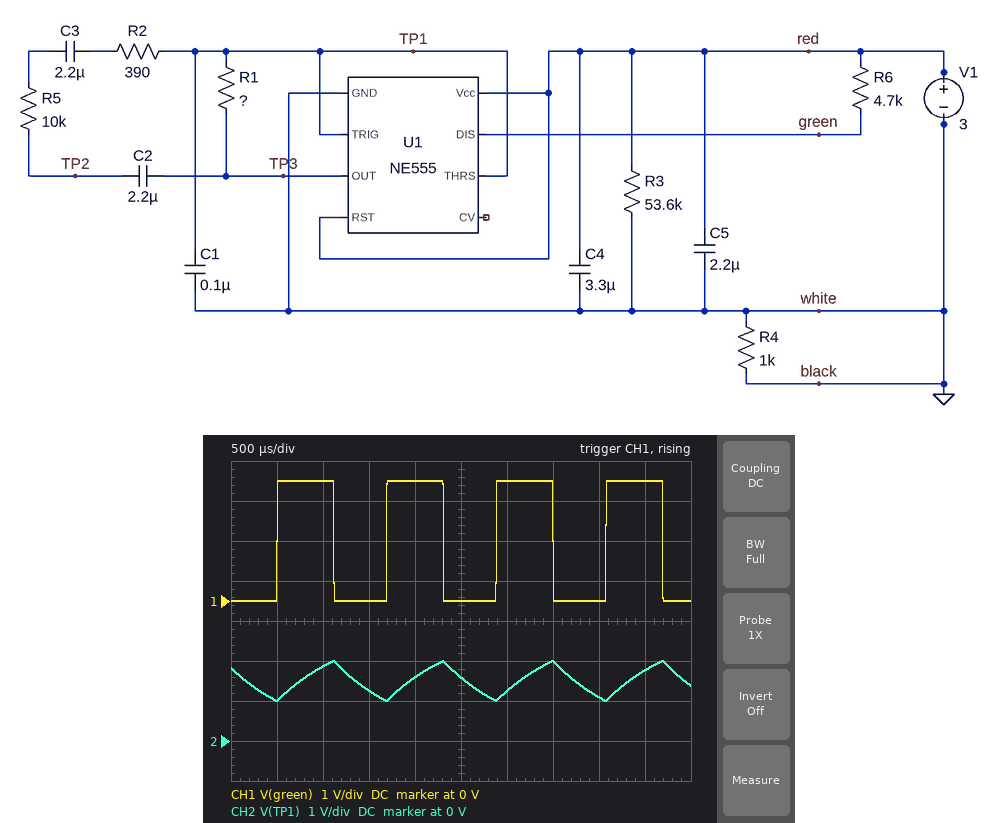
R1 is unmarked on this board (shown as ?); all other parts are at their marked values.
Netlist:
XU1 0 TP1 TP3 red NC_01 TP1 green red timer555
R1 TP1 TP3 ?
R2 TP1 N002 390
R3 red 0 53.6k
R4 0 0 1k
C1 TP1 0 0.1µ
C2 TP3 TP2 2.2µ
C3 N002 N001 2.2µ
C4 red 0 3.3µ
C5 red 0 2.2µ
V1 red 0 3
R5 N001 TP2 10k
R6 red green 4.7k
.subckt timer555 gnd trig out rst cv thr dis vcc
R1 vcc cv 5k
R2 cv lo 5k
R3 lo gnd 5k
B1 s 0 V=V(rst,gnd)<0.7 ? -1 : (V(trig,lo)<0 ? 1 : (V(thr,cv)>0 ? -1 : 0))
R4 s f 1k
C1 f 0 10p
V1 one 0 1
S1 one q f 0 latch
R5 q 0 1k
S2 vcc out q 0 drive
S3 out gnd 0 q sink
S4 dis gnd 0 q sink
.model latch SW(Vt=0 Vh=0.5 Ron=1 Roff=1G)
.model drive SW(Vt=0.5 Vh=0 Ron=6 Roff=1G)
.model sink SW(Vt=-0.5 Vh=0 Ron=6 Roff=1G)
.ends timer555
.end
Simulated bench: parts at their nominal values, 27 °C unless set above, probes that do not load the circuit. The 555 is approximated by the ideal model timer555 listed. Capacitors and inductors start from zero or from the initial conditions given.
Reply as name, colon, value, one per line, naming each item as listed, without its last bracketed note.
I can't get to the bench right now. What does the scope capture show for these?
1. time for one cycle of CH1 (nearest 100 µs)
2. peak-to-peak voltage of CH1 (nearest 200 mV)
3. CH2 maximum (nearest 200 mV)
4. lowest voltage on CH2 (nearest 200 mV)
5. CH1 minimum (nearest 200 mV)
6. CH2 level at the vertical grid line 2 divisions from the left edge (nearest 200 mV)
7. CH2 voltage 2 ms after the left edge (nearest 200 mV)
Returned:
time for one cycle of CH1: 1.2 ms
peak-to-peak voltage of CH1: 3.0 V
CH2 maximum: 2.0 V
lowest voltage on CH2: 1.0 V
CH1 minimum: 0 V
CH2 level at the vertical grid line 2 divisions from the left edge: 1.8 V
CH2 voltage 2 ms after the left edge: 1.6 V
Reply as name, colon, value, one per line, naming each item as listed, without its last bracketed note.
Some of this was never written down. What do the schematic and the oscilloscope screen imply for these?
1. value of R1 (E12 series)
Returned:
value of R1: 47 kΩ
